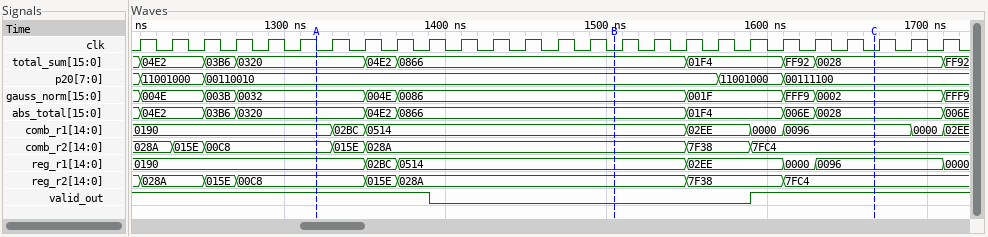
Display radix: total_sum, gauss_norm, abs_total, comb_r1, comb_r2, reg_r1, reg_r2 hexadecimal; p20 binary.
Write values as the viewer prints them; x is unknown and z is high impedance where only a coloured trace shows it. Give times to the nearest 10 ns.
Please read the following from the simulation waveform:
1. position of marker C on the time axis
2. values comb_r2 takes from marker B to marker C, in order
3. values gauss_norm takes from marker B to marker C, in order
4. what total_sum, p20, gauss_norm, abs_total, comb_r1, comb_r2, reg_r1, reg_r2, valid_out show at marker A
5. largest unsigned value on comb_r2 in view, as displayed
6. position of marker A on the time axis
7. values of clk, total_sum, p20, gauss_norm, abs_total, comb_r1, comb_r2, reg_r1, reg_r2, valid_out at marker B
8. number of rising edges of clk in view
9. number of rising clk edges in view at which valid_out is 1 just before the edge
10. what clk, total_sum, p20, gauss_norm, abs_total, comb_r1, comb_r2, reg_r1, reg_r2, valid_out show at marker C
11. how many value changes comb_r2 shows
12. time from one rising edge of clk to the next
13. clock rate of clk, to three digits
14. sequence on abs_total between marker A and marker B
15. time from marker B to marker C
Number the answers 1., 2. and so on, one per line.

1. 1670 ns
2. 028A, 7F38, 7FC4
3. 0086, 001F, FFF9, 0002
4. total_sum=0320, p20=00110010, gauss_norm=0032, abs_total=0320, comb_r1=0190, comb_r2=00C8, reg_r1=0190, reg_r2=00C8, valid_out=1
5. 7FC4
6. 1320 ns
7. clk=0, total_sum=0866, p20=00110010, gauss_norm=0086, abs_total=0866, comb_r1=0514, comb_r2=028A, reg_r1=0514, reg_r2=028A, valid_out=0
8. 26
9. 16
10. clk=0, total_sum=0028, p20=00111100, gauss_norm=0002, abs_total=0028, comb_r1=0096, comb_r2=7FC4, reg_r1=0096, reg_r2=7FC4, valid_out=1
11. 6
12. 20 ns
13. 50.0 MHz
14. 0320, 04E2, 0866
15. 160 ns
